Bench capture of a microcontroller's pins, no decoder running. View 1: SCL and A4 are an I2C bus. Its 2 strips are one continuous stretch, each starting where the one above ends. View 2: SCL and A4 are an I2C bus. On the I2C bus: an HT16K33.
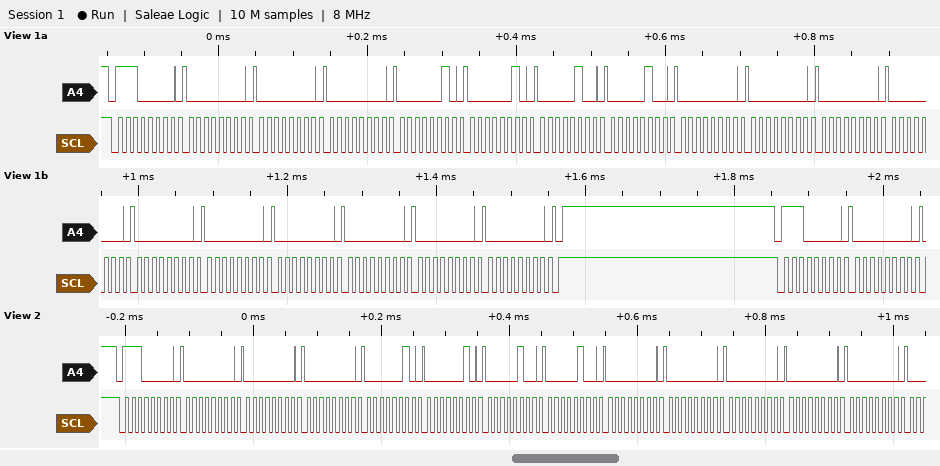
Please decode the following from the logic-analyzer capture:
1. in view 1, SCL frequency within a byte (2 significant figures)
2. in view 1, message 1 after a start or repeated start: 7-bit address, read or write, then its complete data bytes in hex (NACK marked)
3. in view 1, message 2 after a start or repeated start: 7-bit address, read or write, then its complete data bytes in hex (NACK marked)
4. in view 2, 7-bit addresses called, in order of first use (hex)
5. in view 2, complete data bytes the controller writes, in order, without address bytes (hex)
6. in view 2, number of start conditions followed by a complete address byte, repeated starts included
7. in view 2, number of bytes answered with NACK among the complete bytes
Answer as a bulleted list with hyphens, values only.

- 100 kHz
- 0x70 write: 00 00 00 02 02 04 04 00 00 00 00 00 00 00 00 00 00
- 0x70 write: 00
- 0x70
- 00 00 00 02 02 04 04 00 00 00 00 00
- 1
- 0
